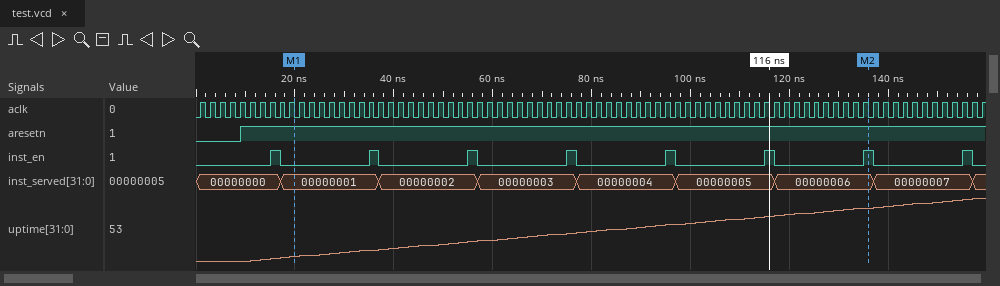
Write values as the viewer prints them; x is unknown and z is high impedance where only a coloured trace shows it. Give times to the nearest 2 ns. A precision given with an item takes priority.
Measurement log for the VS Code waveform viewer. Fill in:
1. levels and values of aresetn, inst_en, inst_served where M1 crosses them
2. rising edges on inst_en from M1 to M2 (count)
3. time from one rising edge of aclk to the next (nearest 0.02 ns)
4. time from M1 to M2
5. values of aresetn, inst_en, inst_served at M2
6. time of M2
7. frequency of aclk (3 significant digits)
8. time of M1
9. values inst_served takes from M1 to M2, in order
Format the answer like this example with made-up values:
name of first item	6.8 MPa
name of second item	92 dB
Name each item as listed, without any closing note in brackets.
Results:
levels and values of aresetn, inst_en, inst_served where M1 crosses them	aresetn=1, inst_en=0, inst_served=00000001
rising edges on inst_en from M1 to M2	6
time from one rising edge of aclk to the next	2 ns
time from M1 to M2	116 ns
values of aresetn, inst_en, inst_served at M2	aresetn=1, inst_en=1, inst_served=00000006
time of M2	136 ns
frequency of aclk	500 MHz
time of M1	20 ns
values inst_served takes from M1 to M2, in order	00000001, 00000002, 00000003, 00000004, 00000005, 00000006
